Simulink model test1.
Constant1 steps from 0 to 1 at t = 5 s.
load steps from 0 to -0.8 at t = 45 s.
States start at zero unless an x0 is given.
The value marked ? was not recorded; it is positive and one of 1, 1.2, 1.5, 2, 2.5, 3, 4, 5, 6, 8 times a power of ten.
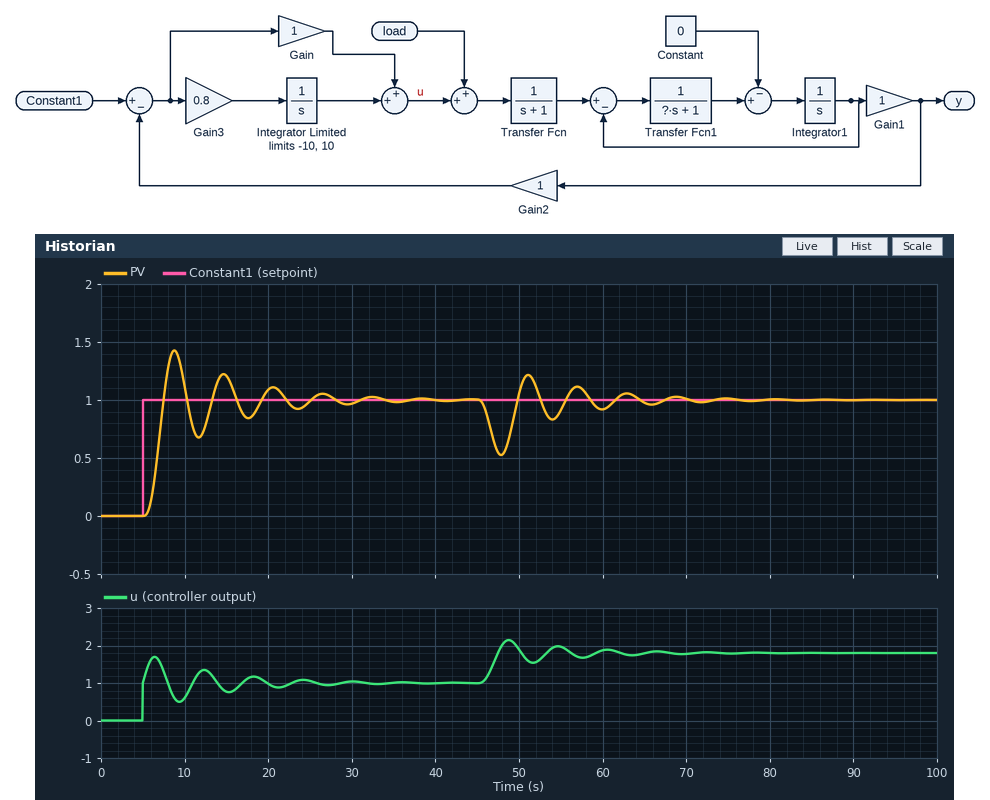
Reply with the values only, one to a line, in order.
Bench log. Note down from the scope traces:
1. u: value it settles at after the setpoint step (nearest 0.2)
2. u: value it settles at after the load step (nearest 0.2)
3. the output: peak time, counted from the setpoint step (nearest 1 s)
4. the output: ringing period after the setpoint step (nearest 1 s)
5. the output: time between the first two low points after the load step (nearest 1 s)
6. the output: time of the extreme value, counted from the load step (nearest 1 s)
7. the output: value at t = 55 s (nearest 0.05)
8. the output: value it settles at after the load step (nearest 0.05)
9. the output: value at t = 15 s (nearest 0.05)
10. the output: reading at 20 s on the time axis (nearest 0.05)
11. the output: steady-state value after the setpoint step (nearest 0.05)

1.0
1.8
4 s
6 s
6 s
3 s
0.90
1.00
1.20
1.10
1.00
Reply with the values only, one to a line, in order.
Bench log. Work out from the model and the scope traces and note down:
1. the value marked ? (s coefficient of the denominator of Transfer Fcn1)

0.8
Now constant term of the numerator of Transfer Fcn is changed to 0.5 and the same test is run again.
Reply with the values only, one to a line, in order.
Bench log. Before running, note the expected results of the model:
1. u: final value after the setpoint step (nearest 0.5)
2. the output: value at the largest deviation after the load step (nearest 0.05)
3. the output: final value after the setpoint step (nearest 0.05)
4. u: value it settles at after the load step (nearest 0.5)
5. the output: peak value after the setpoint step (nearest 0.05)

2.0
0.70
1.00
3.0
1.05
